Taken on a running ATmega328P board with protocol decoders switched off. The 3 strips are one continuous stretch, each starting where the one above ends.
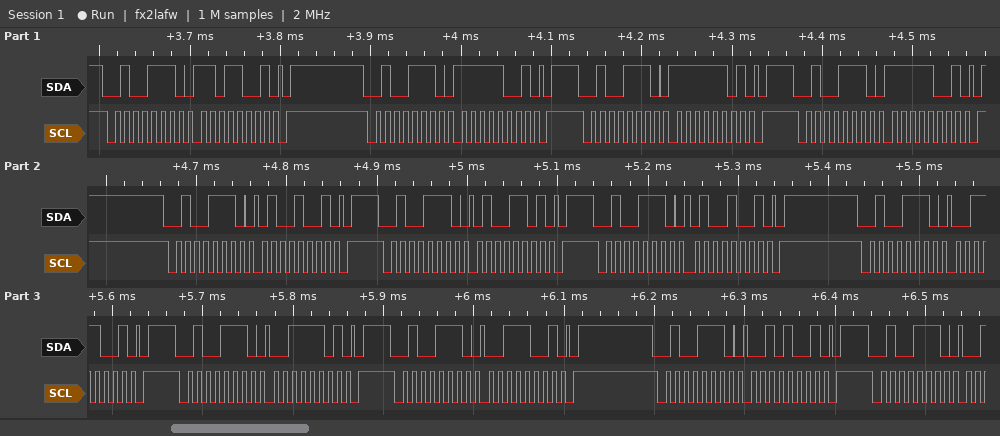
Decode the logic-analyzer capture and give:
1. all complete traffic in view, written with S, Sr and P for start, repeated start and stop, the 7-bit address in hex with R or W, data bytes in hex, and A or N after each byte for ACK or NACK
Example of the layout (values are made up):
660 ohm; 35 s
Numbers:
S 27W A D9 A P S 27W A F9 A P S 27W A FD A P S 27W A F9 A P S 27W A 49 A P S 27W A 4D A P S 27W A 49 A P S 27W A 39 A P S 27W A 3D A P S 27W A 39 A P S 27W A 29 A P S 27W A
